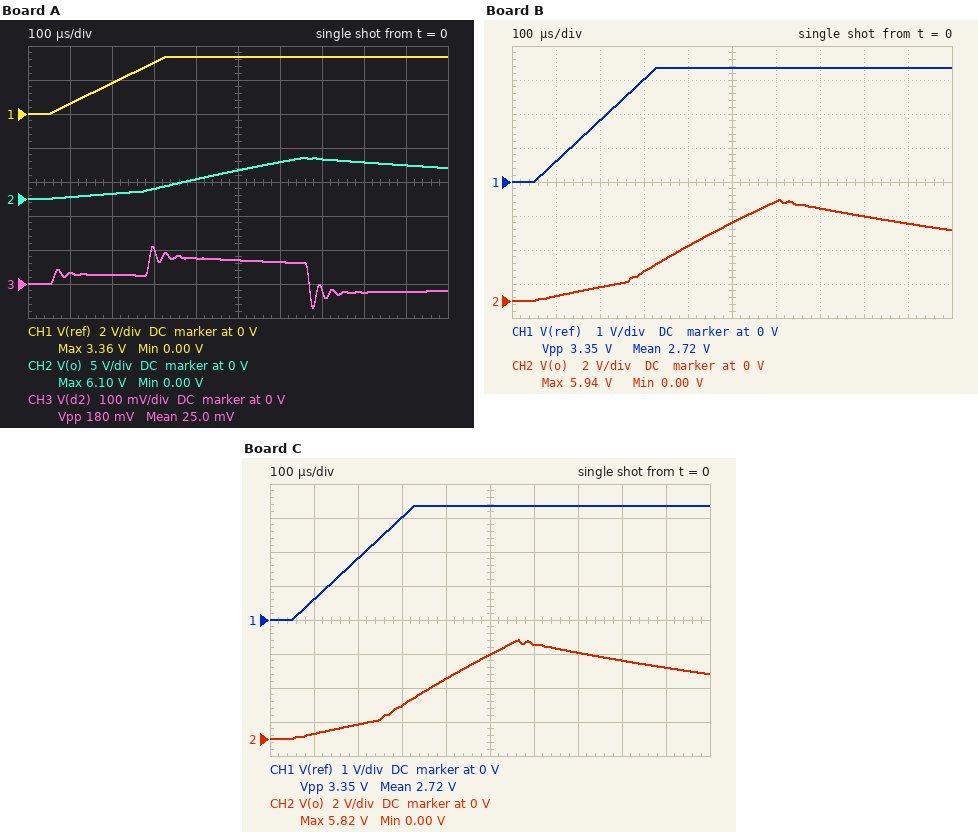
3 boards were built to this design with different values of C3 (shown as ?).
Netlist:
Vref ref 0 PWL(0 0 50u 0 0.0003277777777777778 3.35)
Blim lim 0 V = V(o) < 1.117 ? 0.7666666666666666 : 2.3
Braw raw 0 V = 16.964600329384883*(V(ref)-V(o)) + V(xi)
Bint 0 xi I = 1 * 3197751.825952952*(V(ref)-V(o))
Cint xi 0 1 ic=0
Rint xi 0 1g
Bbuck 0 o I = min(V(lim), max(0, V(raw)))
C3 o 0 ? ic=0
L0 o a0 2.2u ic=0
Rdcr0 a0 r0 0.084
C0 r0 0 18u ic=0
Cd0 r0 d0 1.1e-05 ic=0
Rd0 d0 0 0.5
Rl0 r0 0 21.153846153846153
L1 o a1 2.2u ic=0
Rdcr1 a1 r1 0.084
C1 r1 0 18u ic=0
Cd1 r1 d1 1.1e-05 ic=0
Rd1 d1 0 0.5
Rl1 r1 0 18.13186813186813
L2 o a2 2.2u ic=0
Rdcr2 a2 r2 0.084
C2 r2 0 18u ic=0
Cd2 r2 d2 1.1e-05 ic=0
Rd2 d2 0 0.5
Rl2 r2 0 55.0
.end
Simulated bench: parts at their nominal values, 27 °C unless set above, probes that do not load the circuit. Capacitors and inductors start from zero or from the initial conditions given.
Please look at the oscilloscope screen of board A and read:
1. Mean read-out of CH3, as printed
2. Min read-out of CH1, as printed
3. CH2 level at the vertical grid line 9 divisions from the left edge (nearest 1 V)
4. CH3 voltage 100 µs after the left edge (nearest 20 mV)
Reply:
25.0 mV
0.00 V
5 V
40 mV
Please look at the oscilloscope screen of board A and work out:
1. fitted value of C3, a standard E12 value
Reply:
56 µF
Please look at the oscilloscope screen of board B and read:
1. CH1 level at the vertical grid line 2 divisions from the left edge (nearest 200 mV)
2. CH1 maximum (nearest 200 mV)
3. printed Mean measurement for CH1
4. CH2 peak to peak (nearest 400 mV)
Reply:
1.8 V
3.4 V
2.72 V
6.0 V
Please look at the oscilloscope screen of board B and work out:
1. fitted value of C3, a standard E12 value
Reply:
47 µF
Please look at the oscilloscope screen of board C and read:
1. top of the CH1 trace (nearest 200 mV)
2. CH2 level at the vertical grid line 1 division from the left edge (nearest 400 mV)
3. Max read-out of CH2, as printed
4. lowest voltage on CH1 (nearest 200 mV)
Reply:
3.4 V
400 mV
5.82 V
0 V
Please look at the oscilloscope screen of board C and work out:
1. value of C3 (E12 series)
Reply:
39 µF
